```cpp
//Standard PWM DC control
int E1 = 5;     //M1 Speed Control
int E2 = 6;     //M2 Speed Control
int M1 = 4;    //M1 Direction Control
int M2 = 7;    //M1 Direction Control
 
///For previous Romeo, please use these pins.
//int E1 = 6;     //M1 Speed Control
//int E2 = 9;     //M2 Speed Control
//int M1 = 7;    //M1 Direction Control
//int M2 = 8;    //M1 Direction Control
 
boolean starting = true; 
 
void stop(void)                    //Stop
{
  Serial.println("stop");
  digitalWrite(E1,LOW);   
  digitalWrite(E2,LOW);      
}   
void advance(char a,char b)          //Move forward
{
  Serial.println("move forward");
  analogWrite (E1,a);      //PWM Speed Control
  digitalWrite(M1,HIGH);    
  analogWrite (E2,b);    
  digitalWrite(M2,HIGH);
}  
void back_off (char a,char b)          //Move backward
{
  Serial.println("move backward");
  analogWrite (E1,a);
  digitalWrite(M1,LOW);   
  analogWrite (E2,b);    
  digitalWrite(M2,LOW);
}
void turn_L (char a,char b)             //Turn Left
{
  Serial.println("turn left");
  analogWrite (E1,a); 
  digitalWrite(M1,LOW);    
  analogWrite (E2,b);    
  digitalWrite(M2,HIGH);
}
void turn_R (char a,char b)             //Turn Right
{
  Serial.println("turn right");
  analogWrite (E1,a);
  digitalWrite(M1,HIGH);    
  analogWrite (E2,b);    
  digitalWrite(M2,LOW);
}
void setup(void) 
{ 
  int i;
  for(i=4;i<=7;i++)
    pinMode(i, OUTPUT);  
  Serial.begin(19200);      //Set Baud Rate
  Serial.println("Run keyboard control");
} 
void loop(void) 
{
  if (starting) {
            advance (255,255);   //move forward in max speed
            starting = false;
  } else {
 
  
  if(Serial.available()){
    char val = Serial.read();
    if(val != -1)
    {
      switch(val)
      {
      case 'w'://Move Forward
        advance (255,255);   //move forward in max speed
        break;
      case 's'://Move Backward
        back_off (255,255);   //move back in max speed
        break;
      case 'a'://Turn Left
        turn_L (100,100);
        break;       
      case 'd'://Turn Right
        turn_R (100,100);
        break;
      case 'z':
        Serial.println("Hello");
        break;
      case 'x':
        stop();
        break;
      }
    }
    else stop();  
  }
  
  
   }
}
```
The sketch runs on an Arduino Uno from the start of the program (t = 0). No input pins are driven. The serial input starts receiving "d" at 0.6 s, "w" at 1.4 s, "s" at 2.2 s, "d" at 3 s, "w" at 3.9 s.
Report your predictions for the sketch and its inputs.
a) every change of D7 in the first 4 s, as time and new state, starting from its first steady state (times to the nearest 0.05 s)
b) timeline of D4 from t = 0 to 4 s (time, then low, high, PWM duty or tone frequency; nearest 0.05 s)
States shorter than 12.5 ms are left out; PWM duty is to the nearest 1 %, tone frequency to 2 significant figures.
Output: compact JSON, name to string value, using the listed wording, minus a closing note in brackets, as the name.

{"every change of D7 in the first 4 s, as time and new state, starting from its first steady state": "0 s high; 0.6 s low; 1.4 s high; 2.2 s low; 3.9 s high", "timeline of D4 from t = 0 to 4 s": "0 s high; 2.2 s low; 3 s high"}
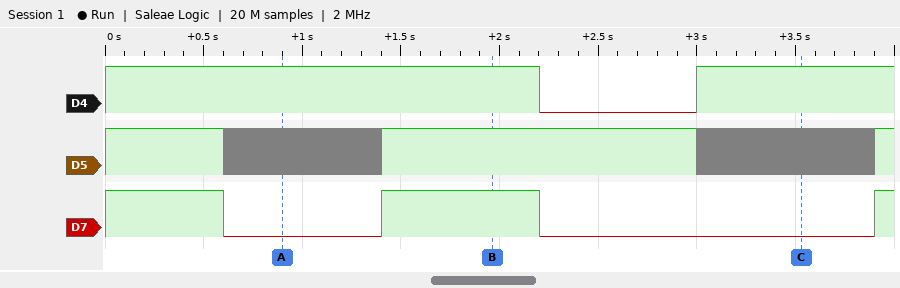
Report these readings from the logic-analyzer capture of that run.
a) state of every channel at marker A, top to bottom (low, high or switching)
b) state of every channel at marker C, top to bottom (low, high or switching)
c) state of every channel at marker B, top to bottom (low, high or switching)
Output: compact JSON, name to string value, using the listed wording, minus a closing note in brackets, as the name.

{"state of every channel at marker A, top to bottom": "D4 high, D5 switching, D7 low", "state of every channel at marker C, top to bottom": "D4 high, D5 switching, D7 low", "state of every channel at marker B, top to bottom": "D4 high, D5 high, D7 high"}
